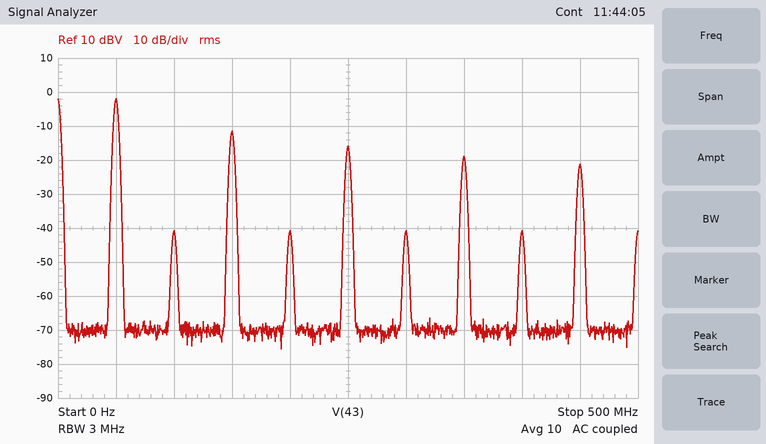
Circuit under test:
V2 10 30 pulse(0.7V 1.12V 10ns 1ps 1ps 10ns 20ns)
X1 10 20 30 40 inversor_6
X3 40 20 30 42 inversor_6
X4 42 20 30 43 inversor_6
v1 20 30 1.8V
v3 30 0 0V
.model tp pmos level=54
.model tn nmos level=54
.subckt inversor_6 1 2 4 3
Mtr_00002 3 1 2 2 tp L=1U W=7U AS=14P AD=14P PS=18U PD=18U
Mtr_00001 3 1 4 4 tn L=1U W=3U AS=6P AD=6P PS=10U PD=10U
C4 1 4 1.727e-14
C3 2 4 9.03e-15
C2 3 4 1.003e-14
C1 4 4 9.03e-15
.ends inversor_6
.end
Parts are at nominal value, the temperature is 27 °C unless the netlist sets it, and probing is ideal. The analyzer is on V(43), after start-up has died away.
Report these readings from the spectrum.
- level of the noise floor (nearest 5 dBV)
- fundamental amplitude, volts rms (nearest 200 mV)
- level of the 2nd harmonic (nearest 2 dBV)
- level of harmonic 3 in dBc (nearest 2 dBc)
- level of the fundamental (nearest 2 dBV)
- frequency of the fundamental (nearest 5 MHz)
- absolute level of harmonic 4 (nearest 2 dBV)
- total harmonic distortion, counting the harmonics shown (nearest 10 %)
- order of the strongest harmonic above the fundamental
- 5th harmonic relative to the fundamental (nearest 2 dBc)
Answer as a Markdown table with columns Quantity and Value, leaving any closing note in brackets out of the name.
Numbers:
| Quantity | Value |
|---|---|
| level of the noise floor | -70 dBV |
| fundamental amplitude, volts rms | 800 mV |
| level of the 2nd harmonic | -40 dBV |
| level of harmonic 3 in dBc | -10 dBc |
| level of the fundamental | -2 dBV |
| frequency of the fundamental | 50 MHz |
| absolute level of harmonic 4 | -40 dBV |
| total harmonic distortion, counting the harmonics shown | 40 % |
| order of the strongest harmonic above the fundamental | 3 |
| 5th harmonic relative to the fundamental | -14 dBc |
